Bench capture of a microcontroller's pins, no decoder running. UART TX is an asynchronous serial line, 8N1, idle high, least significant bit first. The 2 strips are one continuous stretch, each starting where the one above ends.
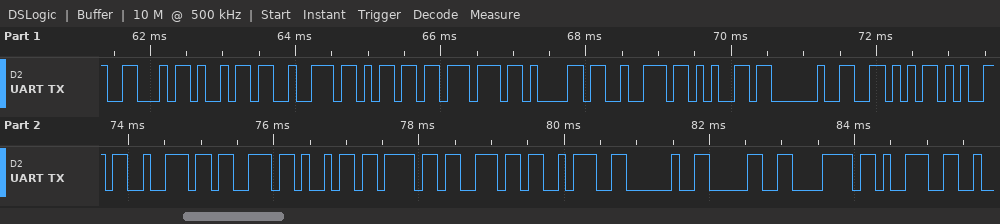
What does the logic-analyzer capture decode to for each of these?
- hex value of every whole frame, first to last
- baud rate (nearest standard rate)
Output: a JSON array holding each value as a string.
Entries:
["46 69 72 6D 77 61 72 65 20 56 65 72 73 69 6F 6E 3A 20 30 78 39", "9600 baud"]
